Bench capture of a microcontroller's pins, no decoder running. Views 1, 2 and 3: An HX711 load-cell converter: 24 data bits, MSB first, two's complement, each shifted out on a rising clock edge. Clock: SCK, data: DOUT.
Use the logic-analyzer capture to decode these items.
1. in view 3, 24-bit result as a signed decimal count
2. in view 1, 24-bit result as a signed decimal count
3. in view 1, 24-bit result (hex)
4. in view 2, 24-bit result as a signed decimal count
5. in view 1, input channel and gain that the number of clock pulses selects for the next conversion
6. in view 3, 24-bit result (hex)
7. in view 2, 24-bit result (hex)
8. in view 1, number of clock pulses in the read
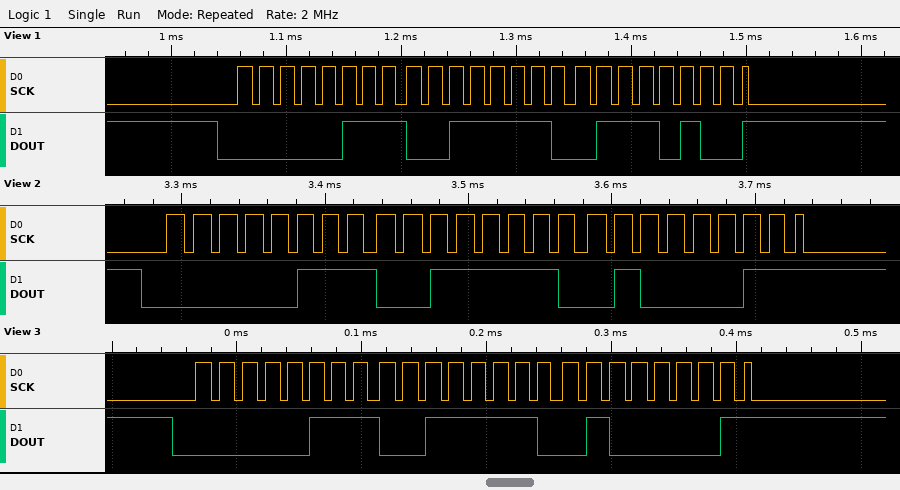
474689
474740
0x073E74
474691
channel A, gain 128
0x073E41
0x073E43
25
